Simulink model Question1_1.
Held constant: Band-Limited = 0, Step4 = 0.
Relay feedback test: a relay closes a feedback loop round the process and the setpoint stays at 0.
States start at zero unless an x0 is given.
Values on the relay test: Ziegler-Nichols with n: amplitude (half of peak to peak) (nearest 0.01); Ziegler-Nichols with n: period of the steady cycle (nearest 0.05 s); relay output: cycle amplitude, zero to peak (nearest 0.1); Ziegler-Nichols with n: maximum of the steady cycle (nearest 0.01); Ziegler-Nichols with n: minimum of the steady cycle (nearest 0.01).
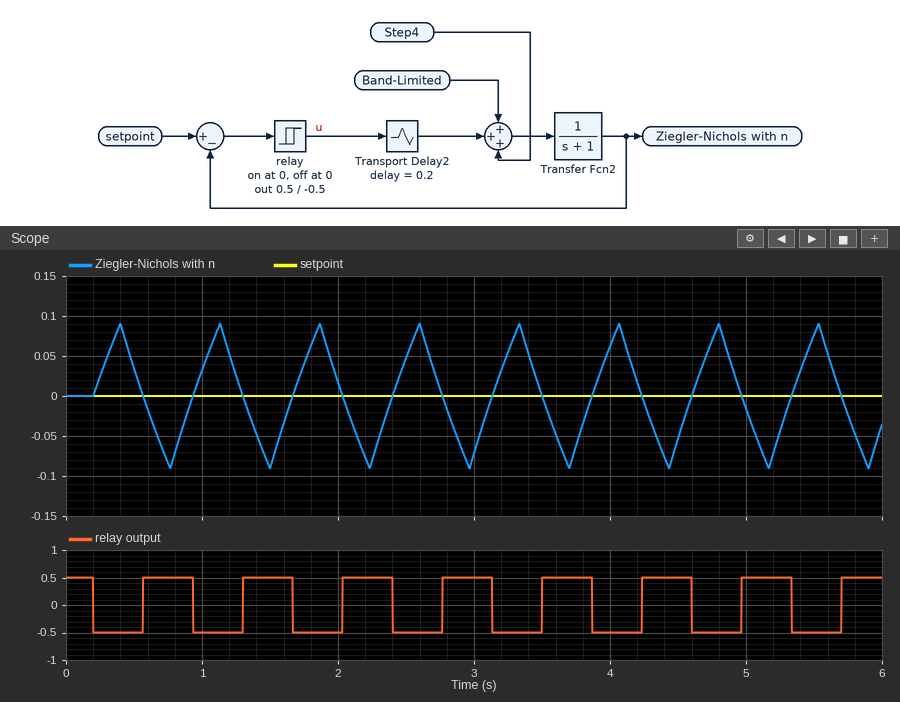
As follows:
0.09
0.75 s
0.5
0.09
-0.09
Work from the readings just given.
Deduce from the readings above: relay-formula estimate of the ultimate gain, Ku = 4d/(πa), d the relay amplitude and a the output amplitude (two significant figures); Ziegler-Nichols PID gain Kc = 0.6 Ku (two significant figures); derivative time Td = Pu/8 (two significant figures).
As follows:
7.1
4.3
0.094 s
